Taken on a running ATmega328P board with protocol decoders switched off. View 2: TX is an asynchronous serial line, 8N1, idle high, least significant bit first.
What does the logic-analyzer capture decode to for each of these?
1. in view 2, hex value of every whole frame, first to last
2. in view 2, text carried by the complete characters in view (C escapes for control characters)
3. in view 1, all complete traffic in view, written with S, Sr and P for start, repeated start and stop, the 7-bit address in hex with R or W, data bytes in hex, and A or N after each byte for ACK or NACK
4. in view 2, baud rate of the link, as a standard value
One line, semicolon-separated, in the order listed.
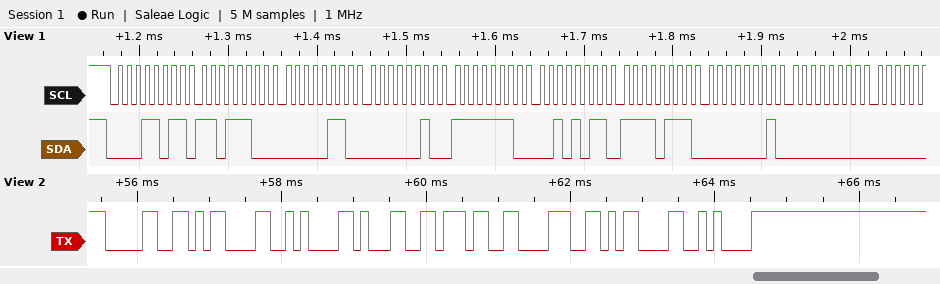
30 0D 0A 31 37 38 0D 0A; "0\r\n178\r\n"; S 0DR A DC A 06 A 02 A FE A 2B A F7 A 01 A 00 A; 9600 baud
